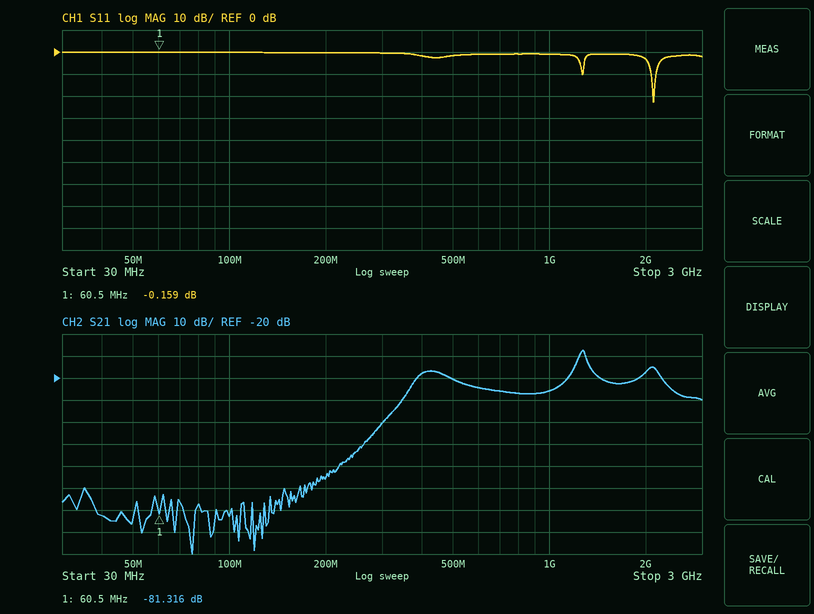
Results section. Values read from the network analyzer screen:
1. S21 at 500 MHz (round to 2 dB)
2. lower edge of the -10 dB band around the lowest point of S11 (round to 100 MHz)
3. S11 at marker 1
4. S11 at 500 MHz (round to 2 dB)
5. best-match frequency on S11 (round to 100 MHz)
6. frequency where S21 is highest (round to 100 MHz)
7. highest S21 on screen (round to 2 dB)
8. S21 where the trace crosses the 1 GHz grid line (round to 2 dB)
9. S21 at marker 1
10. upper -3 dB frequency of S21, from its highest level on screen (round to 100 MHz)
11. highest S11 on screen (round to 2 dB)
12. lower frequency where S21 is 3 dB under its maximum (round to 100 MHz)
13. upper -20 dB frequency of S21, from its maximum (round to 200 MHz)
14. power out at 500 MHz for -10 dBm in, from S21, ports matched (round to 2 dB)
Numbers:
-20 dB
2.1 GHz
-0.159 dB
-2 dB
2.1 GHz
1.3 GHz
-8 dB
-26 dB
-81.316 dB
1.3 GHz
0 dB
1.2 GHz
2.6 GHz
-30 dBm
